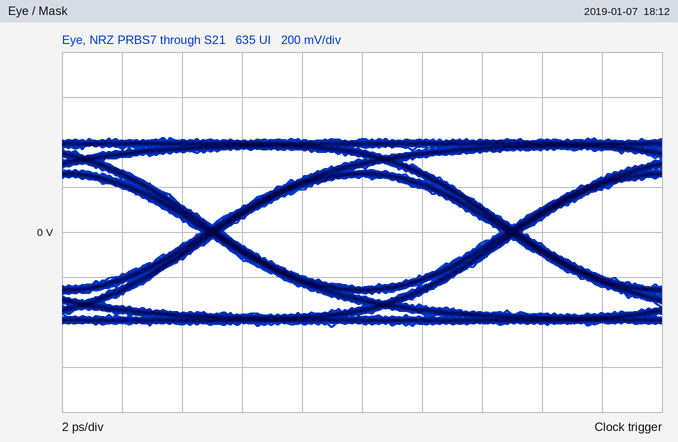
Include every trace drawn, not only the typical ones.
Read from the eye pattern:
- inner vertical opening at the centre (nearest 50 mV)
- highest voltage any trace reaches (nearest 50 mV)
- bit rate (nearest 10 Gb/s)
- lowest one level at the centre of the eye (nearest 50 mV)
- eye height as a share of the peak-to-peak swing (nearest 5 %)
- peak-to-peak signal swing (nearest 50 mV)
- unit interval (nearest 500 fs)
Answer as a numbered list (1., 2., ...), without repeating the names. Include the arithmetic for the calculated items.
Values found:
1. 500 mV
2. 400 mV
3. 100 Gb/s
4. 250 mV
5. 500 mV / 850 mV ≈ 58.8 %, so 60 % to the nearest 5 %
6. 850 mV
7. 10.0 ps
